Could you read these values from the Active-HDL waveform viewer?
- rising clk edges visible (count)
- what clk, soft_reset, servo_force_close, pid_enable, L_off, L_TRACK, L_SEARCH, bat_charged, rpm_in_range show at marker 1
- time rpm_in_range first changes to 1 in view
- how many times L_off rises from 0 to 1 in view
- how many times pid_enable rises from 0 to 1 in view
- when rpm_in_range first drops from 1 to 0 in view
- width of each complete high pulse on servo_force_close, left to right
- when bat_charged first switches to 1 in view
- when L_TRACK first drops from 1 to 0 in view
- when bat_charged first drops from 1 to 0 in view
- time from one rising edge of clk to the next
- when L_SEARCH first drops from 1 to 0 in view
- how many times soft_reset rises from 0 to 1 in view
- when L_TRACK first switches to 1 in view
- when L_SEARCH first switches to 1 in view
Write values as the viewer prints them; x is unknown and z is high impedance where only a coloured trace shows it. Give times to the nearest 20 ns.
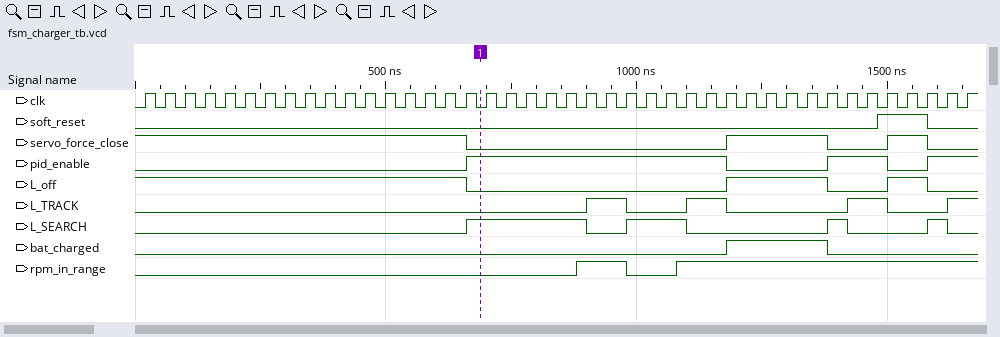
42
clk=0, soft_reset=0, servo_force_close=0, pid_enable=1, L_off=0, L_TRACK=0, L_SEARCH=1, bat_charged=0, rpm_in_range=0
880 ns
2
3
980 ns
200 ns, 80 ns
1180 ns
980 ns
1380 ns
40 ns
900 ns
1
900 ns
660 ns
